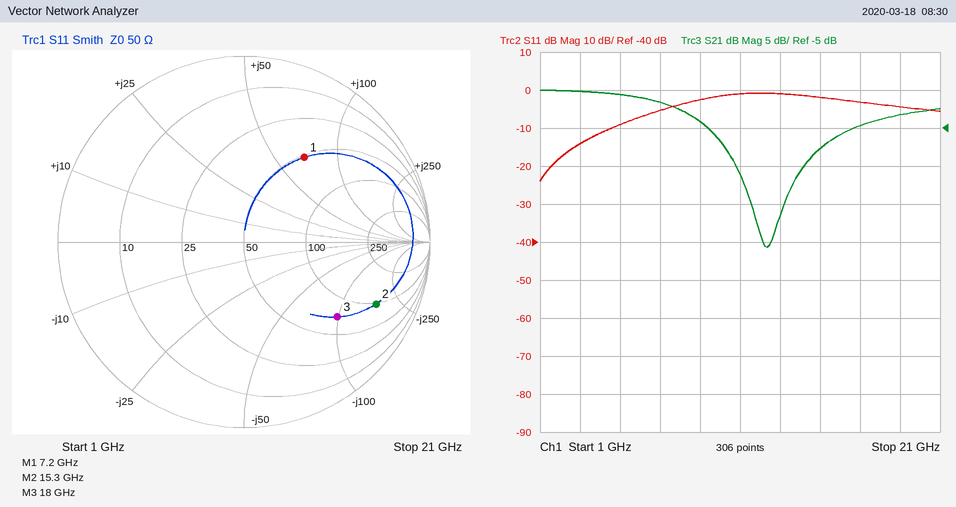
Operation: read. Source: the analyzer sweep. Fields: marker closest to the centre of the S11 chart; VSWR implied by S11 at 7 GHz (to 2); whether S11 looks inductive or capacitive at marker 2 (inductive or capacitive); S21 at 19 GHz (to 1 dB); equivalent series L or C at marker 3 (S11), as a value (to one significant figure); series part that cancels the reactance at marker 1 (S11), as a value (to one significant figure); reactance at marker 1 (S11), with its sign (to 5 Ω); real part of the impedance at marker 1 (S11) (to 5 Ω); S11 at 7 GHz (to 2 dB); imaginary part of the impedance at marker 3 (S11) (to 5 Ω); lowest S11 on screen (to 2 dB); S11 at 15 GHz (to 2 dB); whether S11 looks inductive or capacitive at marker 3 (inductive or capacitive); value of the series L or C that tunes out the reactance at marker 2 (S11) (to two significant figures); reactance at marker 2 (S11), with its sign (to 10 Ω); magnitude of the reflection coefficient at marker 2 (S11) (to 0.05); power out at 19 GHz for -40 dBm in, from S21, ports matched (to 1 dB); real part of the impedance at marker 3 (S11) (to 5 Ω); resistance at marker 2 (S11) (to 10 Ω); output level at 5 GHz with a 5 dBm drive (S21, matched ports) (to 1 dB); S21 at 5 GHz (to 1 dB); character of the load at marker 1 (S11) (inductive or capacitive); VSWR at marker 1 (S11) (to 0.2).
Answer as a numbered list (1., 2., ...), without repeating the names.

1. marker 1
2. 4
3. capacitive
4. -3 dB
5. 90 fF
6. 300 fF
7. +70 Ω
8. 50 Ω
9. -6 dB
10. -100 Ω
11. -24 dB
12. -2 dB
13. capacitive
14. 1.8 nH
15. -170 Ω
16. 0.80
17. -43 dBm
18. 70 Ω
19. 100 Ω
20. 4 dBm
21. -1 dB
22. inductive
23. 3.6
